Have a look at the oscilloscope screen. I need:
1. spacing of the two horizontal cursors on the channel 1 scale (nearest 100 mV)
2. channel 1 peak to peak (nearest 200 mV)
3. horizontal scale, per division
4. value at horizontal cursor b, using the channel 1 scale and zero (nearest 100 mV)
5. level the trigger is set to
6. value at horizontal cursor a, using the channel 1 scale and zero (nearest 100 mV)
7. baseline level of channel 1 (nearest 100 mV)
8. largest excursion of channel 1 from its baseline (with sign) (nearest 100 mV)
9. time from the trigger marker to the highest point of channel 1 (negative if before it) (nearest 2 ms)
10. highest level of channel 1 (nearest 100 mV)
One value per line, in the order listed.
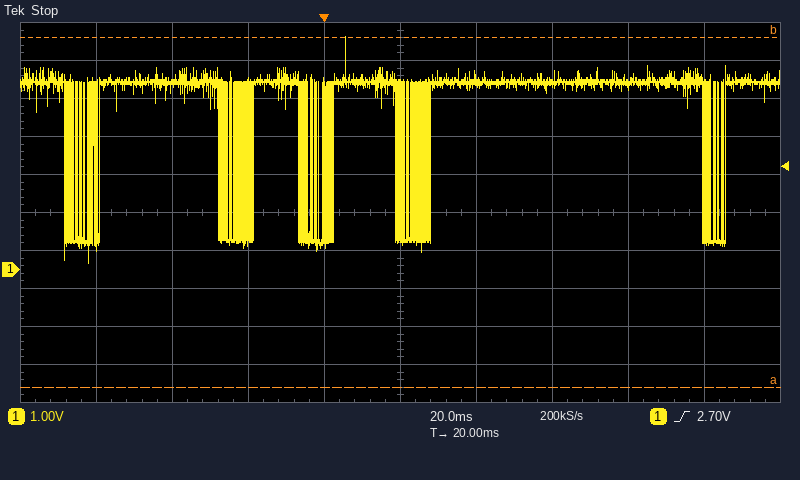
9.2 V
6.0 V
20 ms
6.1 V
2.70 V
-3.1 V
4.9 V
-4.8 V
+6 ms
6.1 V
